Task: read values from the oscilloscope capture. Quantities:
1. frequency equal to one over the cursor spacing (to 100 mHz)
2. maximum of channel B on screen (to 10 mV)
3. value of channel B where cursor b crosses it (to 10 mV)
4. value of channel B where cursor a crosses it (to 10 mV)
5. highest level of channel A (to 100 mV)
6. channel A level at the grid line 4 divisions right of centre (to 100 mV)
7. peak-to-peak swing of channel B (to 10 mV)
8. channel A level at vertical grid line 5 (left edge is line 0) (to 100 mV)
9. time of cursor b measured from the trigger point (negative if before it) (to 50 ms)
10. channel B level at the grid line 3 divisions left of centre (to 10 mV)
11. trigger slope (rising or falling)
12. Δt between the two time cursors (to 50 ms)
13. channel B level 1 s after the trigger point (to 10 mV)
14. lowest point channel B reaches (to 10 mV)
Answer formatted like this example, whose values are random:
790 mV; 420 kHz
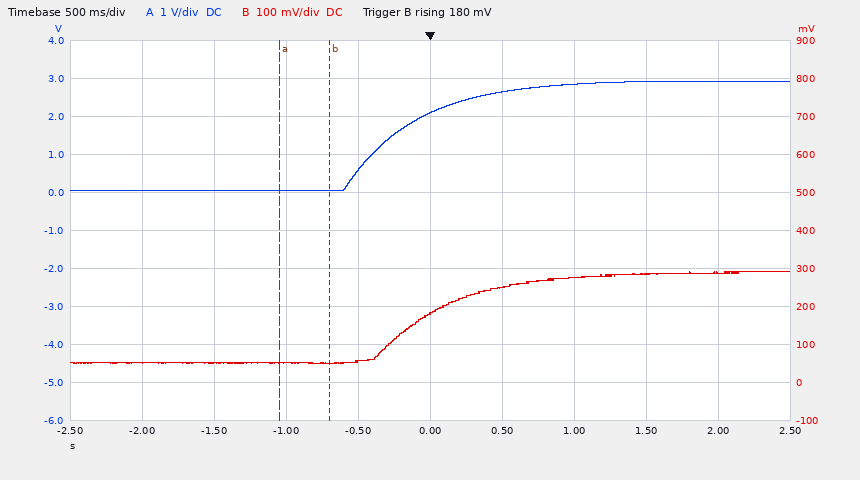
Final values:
2.9 Hz; 290 mV; 50 mV; 50 mV; 2.9 V; 2.9 V; 240 mV; 2.1 V; -700 ms; 50 mV; rising; 350 ms; 280 mV; 50 mV
